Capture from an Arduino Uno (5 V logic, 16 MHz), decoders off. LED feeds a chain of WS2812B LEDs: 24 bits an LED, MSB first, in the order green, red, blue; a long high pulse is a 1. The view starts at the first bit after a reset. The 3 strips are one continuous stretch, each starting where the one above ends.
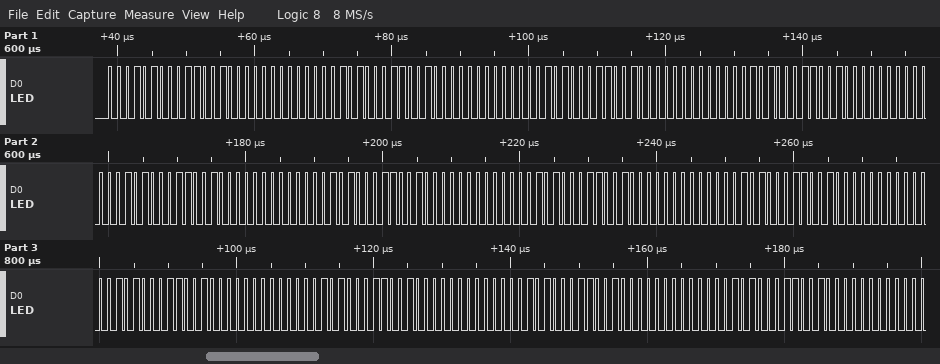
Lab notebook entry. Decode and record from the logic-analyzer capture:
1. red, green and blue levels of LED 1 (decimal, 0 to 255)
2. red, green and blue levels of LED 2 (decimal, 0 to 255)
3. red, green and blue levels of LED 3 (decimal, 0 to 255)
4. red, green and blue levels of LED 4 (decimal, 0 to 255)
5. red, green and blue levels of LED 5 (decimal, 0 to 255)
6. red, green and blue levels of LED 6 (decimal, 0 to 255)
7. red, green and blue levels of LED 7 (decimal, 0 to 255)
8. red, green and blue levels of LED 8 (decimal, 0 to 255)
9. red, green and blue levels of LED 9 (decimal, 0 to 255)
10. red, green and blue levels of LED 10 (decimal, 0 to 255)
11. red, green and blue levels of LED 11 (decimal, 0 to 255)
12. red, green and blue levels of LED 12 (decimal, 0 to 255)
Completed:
100, 20, 0
100, 20, 0
100, 20, 0
100, 20, 0
100, 20, 0
100, 20, 0
100, 20, 0
100, 20, 0
100, 20, 0
100, 20, 0
100, 20, 0
100, 20, 0
